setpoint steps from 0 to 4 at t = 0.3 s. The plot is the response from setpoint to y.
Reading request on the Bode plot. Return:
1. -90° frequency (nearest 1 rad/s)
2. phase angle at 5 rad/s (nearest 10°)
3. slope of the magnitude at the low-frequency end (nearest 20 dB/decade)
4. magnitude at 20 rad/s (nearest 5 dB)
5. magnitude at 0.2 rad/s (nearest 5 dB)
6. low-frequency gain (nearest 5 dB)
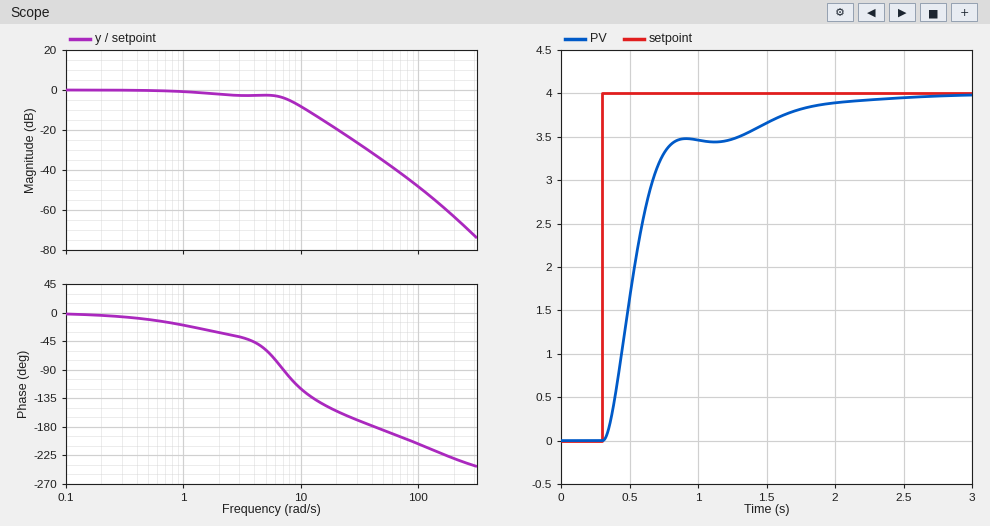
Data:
7 rad/s
-60°
0 dB/decade
-20 dB
0 dB
0 dB
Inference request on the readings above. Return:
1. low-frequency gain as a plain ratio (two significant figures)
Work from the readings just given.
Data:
1.0
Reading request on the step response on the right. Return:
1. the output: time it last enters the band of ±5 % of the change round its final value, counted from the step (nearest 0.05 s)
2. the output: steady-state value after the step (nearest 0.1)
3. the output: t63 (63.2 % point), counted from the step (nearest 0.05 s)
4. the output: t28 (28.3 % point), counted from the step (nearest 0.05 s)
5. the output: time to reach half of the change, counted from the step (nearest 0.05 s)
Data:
1.40 s
4.0
0.30 s
0.15 s
0.25 s
